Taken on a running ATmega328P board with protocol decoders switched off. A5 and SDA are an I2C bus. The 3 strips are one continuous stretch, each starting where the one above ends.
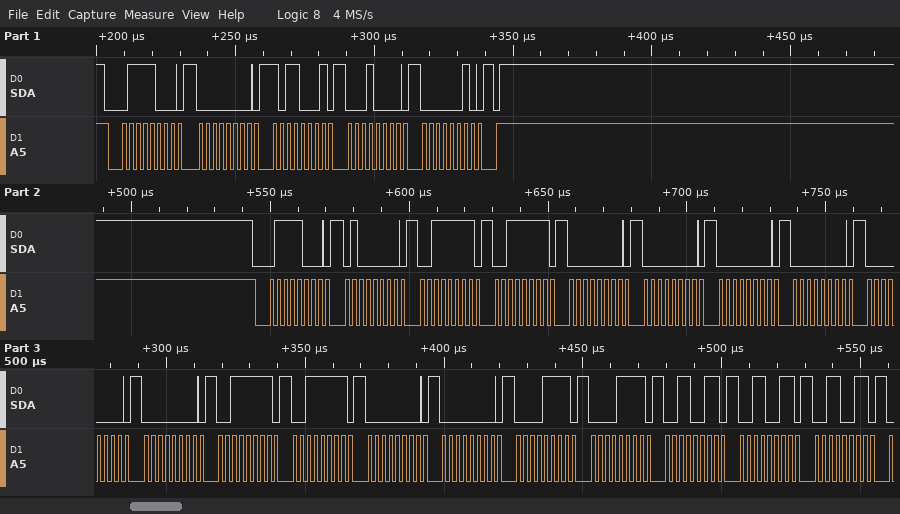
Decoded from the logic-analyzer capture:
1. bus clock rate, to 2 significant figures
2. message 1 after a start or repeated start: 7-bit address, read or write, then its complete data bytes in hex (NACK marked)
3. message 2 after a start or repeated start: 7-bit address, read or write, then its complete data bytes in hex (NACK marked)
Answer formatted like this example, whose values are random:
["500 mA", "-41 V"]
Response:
["400 kHz", "0x3C write: 00 B1 10 02", "0x3C write: 40 3F 3F 00 00 00 00 00 00 3F 3F 00 00 0F 0F 33 33 33"]
